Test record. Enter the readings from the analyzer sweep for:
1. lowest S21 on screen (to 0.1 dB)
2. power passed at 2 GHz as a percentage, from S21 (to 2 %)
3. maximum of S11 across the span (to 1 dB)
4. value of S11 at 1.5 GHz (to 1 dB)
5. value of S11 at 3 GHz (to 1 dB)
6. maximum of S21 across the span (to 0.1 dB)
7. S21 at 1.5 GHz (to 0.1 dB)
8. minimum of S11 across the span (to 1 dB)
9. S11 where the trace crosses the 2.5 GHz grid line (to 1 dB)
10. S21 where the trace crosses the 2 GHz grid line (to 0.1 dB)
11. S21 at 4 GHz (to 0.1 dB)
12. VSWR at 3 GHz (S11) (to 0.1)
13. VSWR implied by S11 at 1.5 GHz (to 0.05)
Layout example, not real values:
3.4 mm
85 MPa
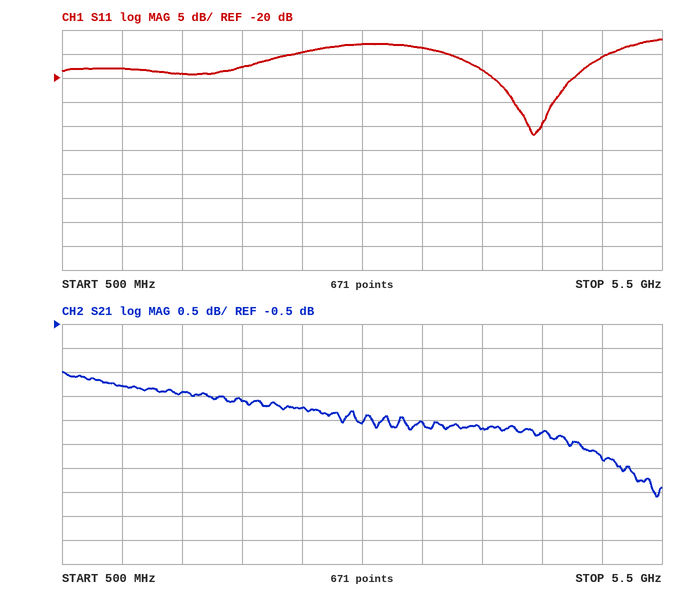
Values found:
-4.1 dB
62 %
-12 dB
-19 dB
-13 dB
-1.5 dB
-1.9 dB
-32 dB
-15 dB
-2.1 dB
-2.7 dB
1.6
1.25
